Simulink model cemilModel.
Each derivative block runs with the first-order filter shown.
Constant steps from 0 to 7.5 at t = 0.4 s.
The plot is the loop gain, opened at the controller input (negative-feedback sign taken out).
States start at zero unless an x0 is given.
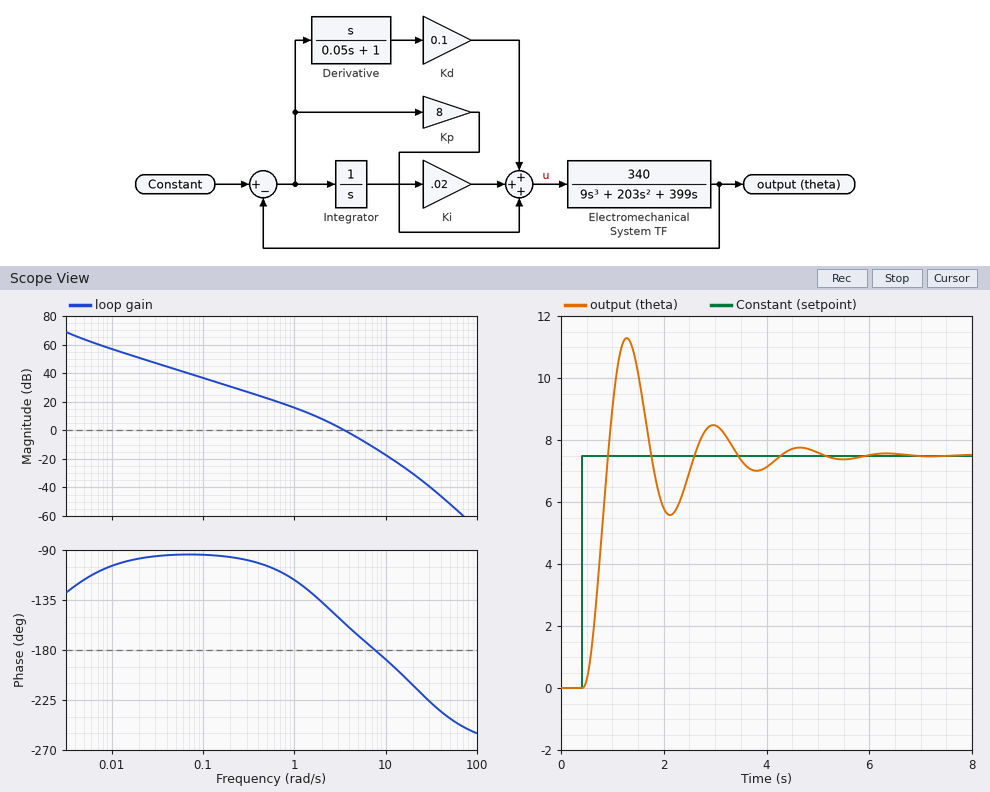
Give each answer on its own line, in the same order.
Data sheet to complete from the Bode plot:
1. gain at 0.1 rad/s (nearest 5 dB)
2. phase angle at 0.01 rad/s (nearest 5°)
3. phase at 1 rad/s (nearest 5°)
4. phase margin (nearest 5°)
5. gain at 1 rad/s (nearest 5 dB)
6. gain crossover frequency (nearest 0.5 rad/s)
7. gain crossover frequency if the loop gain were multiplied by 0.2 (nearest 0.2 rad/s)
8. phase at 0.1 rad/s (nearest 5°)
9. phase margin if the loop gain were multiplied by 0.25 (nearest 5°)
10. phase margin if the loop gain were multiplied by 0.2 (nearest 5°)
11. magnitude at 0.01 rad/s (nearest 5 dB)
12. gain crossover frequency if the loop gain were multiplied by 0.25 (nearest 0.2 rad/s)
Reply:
35 dB
-105°
-115°
25°
15 dB
3.5 rad/s
1.2 rad/s
-95°
55°
60°
55 dB
1.4 rad/s
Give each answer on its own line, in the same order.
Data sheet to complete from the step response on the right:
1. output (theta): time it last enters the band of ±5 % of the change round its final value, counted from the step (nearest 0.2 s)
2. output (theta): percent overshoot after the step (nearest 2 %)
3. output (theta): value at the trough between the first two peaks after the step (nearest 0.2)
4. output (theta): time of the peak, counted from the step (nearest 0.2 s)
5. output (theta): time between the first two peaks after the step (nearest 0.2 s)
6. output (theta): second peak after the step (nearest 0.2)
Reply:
3.6 s
50 %
5.6
0.8 s
1.6 s
8.4
